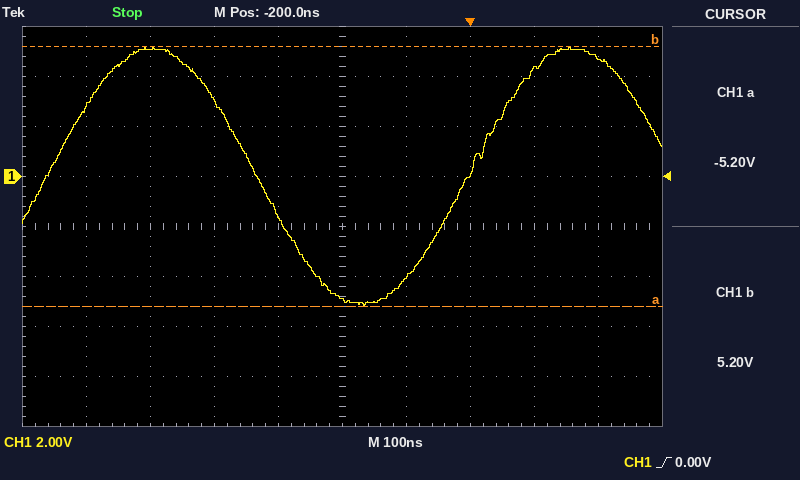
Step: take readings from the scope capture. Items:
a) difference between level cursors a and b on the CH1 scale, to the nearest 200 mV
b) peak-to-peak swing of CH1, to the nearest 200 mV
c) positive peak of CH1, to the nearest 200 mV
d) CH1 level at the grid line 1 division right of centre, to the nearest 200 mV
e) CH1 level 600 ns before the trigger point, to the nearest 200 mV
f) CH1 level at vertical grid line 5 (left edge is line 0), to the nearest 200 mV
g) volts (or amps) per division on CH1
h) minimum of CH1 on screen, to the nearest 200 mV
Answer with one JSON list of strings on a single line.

["10.4 V", "10.4 V", "5.2 V", "-4.0 V", "2.8 V", "-5.0 V", "2 V", "-5.2 V"]
